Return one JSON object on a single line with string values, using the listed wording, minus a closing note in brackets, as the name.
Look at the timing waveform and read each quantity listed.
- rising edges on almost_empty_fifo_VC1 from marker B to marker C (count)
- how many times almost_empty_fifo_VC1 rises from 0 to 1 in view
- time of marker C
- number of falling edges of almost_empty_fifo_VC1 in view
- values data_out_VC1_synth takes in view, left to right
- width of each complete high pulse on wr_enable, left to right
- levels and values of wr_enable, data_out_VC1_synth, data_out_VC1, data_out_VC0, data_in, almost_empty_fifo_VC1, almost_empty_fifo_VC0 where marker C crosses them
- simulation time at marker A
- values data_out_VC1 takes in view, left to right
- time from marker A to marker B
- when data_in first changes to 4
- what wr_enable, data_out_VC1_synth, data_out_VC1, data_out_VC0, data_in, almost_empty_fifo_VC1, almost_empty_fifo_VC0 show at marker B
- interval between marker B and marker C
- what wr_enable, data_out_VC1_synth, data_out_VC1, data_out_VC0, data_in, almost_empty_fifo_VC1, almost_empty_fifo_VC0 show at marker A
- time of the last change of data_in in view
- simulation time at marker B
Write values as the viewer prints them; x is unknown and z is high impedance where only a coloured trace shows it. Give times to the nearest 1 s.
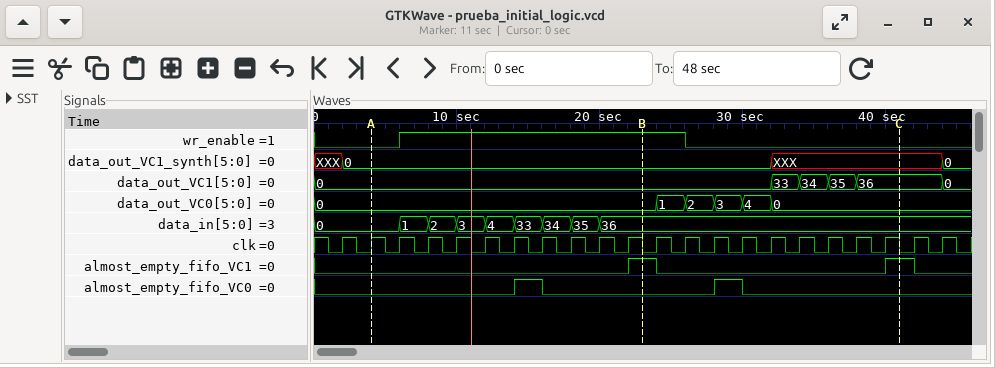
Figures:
{"rising edges on almost_empty_fifo_VC1 from marker B to marker C": "1", "how many times almost_empty_fifo_VC1 rises from 0 to 1 in view": "2", "time of marker C": "41 s", "number of falling edges of almost_empty_fifo_VC1 in view": "2", "values data_out_VC1_synth takes in view, left to right": "XXX, 0, XXX, 0", "width of each complete high pulse on wr_enable, left to right": "20 s", "levels and values of wr_enable, data_out_VC1_synth, data_out_VC1, data_out_VC0, data_in, almost_empty_fifo_VC1, almost_empty_fifo_VC0 where marker C crosses them": "wr_enable=0, data_out_VC1_synth=XXX, data_out_VC1=36, data_out_VC0=0, data_in=36, almost_empty_fifo_VC1=1, almost_empty_fifo_VC0=0", "simulation time at marker A": "4 s", "values data_out_VC1 takes in view, left to right": "0, 33, 34, 35, 36, 0", "time from marker A to marker B": "19 s", "when data_in first changes to 4": "12 s", "what wr_enable, data_out_VC1_synth, data_out_VC1, data_out_VC0, data_in, almost_empty_fifo_VC1, almost_empty_fifo_VC0 show at marker B": "wr_enable=1, data_out_VC1_synth=0, data_out_VC1=0, data_out_VC0=0, data_in=36, almost_empty_fifo_VC1=1, almost_empty_fifo_VC0=0", "interval between marker B and marker C": "18 s", "what wr_enable, data_out_VC1_synth, data_out_VC1, data_out_VC0, data_in, almost_empty_fifo_VC1, almost_empty_fifo_VC0 show at marker A": "wr_enable=0, data_out_VC1_synth=0, data_out_VC1=0, data_out_VC0=0, data_in=0, almost_empty_fifo_VC1=0, almost_empty_fifo_VC0=0", "time of the last change of data_in in view": "20 s", "simulation time at marker B": "23 s"}
